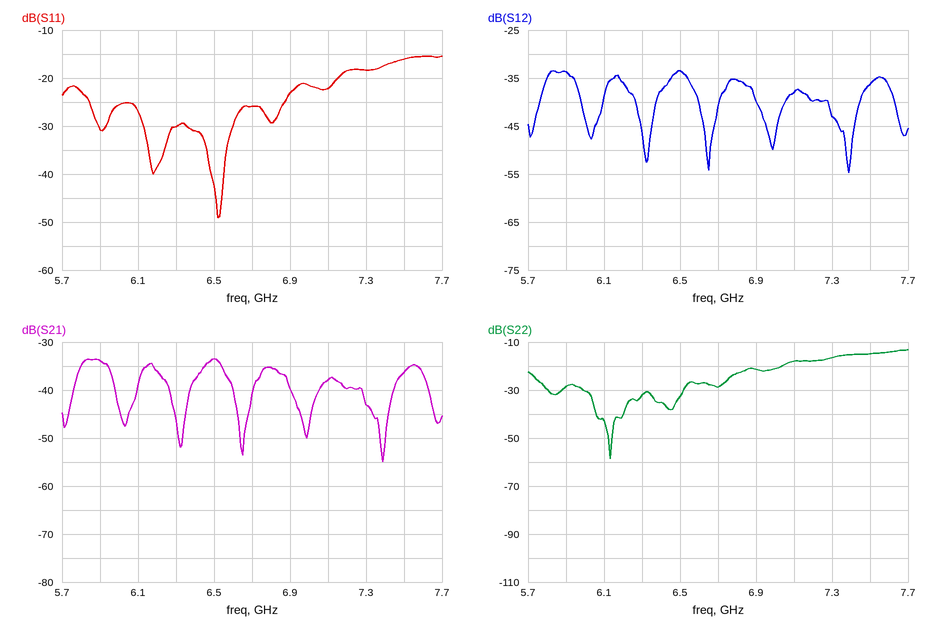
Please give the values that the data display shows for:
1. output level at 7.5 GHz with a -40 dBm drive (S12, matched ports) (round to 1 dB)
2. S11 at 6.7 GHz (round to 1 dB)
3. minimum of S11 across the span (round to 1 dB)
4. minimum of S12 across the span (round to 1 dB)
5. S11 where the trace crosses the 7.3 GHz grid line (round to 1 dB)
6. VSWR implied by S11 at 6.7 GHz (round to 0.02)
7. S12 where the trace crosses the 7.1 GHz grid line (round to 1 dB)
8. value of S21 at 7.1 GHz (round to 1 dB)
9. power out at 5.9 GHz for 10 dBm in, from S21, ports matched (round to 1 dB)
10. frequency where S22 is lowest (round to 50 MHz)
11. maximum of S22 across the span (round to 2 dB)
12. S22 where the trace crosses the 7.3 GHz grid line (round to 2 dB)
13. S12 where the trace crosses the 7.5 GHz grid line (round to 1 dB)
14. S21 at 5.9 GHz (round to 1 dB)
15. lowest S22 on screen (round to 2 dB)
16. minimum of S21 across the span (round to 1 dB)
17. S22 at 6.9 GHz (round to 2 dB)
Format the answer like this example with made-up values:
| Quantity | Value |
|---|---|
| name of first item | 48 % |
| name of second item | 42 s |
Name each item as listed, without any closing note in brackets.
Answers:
| Quantity | Value |
|---|---|
| output level at 7.5 GHz with a -40 dBm drive (S12, matched ports) | -76 dBm |
| S11 at 6.7 GHz | -26 dB |
| minimum of S11 across the span | -49 dB |
| minimum of S12 across the span | -55 dB |
| S11 where the trace crosses the 7.3 GHz grid line | -18 dB |
| VSWR implied by S11 at 6.7 GHz | 1.10 |
| S12 where the trace crosses the 7.1 GHz grid line | -38 dB |
| value of S21 at 7.1 GHz | -38 dB |
| power out at 5.9 GHz for 10 dBm in, from S21, ports matched | -24 dBm |
| frequency where S22 is lowest | 6.15 GHz |
| maximum of S22 across the span | -14 dB |
| S22 where the trace crosses the 7.3 GHz grid line | -16 dB |
| S12 where the trace crosses the 7.5 GHz grid line | -36 dB |
| S21 at 5.9 GHz | -34 dB |
| lowest S22 on screen | -58 dB |
| minimum of S21 across the span | -55 dB |
| S22 at 6.9 GHz | -22 dB |
